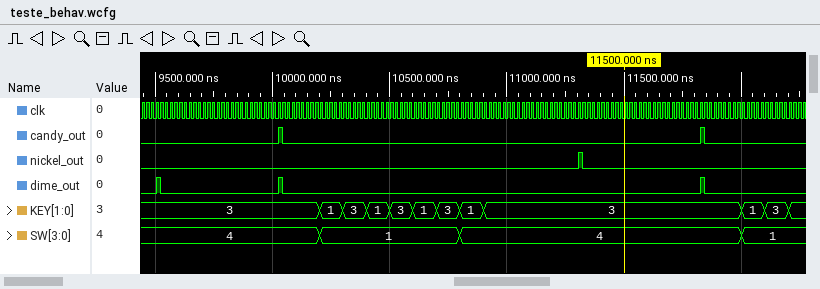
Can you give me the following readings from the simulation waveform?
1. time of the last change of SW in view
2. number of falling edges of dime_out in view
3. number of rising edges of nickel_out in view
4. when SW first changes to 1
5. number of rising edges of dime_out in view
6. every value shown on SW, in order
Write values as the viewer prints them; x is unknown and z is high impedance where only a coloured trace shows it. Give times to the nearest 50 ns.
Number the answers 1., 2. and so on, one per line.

1. 12000 ns
2. 3
3. 1
4. 10200 ns
5. 3
6. 4, 1, 4, 1
